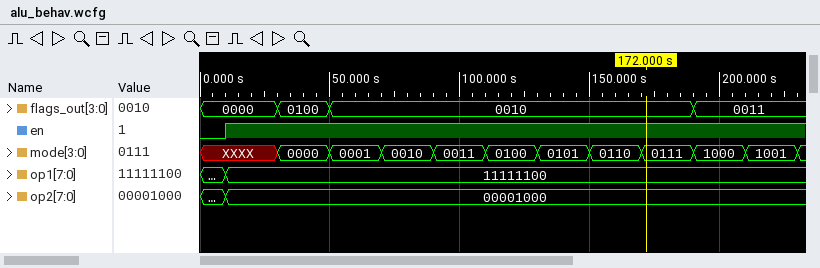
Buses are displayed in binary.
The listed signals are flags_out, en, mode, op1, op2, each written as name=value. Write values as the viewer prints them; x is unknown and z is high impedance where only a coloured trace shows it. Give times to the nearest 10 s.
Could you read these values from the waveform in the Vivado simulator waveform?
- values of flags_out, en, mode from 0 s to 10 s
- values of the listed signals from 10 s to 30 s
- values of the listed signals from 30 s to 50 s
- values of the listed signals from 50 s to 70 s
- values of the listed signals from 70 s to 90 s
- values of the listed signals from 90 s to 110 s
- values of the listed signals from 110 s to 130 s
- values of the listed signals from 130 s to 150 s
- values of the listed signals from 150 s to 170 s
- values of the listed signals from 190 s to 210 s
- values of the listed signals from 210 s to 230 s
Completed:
flags_out=0000, en=0, mode=XXXX
flags_out=0000, en=1, mode=XXXX, op1=11111100, op2=00001000
flags_out=0100, en=1, mode=0000, op1=11111100, op2=00001000
flags_out=0010, en=1, mode=0001, op1=11111100, op2=00001000
flags_out=0010, en=1, mode=0010, op1=11111100, op2=00001000
flags_out=0010, en=1, mode=0011, op1=11111100, op2=00001000
flags_out=0010, en=1, mode=0100, op1=11111100, op2=00001000
flags_out=0010, en=1, mode=0101, op1=11111100, op2=00001000
flags_out=0010, en=1, mode=0110, op1=11111100, op2=00001000
flags_out=0011, en=1, mode=1000, op1=11111100, op2=00001000
flags_out=0011, en=1, mode=1001, op1=11111100, op2=00001000
